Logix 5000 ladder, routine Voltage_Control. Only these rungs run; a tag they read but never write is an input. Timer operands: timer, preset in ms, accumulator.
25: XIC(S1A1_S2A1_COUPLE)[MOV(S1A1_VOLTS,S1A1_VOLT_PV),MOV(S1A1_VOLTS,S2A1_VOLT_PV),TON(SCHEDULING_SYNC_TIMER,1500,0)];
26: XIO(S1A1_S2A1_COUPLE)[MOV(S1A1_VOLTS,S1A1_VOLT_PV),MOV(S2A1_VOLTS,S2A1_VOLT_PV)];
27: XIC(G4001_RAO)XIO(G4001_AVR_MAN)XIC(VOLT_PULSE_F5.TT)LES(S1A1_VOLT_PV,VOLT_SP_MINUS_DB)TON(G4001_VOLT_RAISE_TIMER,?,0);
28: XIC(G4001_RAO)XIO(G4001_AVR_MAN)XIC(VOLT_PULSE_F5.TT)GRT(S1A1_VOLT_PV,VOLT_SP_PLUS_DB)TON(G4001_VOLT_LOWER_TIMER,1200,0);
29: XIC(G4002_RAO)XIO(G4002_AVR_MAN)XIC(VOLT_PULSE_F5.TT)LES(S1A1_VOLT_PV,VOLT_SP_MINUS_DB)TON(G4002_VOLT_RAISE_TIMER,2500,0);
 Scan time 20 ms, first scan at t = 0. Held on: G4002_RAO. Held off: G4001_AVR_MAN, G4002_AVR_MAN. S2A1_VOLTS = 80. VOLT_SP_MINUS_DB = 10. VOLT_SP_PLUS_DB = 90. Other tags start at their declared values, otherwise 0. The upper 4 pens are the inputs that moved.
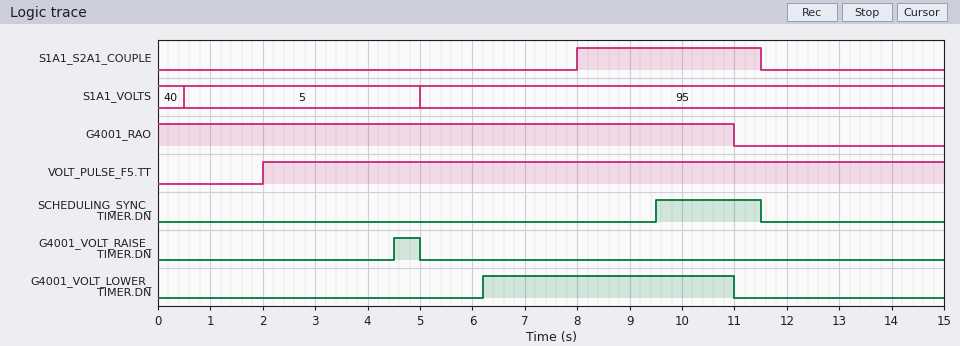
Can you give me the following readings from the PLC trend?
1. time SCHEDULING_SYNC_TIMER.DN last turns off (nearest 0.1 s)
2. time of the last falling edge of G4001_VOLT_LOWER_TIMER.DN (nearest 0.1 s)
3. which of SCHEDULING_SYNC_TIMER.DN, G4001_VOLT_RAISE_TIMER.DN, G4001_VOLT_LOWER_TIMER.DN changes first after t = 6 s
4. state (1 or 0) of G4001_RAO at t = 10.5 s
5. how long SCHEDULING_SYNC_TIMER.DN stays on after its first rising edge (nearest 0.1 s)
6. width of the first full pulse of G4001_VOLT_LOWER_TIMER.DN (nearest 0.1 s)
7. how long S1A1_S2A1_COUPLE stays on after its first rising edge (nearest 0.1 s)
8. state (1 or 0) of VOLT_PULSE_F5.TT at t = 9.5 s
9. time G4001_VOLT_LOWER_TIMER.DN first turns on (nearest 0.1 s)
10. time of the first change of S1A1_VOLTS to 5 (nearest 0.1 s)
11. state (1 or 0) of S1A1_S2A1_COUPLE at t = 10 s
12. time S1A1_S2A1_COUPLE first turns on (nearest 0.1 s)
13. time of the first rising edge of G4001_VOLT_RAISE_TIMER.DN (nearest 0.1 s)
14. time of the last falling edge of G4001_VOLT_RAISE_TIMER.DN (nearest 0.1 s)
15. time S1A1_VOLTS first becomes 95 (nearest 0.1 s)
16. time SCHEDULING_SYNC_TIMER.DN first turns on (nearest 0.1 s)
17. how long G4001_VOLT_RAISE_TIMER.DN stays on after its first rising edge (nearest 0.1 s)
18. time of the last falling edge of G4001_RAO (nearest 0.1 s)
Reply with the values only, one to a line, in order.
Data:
11.5 s
11.0 s
G4001_VOLT_LOWER_TIMER.DN
1
2.0 s
4.8 s
3.5 s
1
6.2 s
0.5 s
1
8.0 s
4.5 s
5.0 s
5.0 s
9.5 s
0.5 s
11.0 s
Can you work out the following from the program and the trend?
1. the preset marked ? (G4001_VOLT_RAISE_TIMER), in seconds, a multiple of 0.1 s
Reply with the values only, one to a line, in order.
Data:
2.5 s
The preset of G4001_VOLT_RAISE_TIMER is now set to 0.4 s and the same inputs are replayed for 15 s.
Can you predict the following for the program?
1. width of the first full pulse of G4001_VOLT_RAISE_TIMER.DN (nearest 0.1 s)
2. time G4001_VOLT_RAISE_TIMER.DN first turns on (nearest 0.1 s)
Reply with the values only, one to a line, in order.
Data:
2.6 s
2.4 s
